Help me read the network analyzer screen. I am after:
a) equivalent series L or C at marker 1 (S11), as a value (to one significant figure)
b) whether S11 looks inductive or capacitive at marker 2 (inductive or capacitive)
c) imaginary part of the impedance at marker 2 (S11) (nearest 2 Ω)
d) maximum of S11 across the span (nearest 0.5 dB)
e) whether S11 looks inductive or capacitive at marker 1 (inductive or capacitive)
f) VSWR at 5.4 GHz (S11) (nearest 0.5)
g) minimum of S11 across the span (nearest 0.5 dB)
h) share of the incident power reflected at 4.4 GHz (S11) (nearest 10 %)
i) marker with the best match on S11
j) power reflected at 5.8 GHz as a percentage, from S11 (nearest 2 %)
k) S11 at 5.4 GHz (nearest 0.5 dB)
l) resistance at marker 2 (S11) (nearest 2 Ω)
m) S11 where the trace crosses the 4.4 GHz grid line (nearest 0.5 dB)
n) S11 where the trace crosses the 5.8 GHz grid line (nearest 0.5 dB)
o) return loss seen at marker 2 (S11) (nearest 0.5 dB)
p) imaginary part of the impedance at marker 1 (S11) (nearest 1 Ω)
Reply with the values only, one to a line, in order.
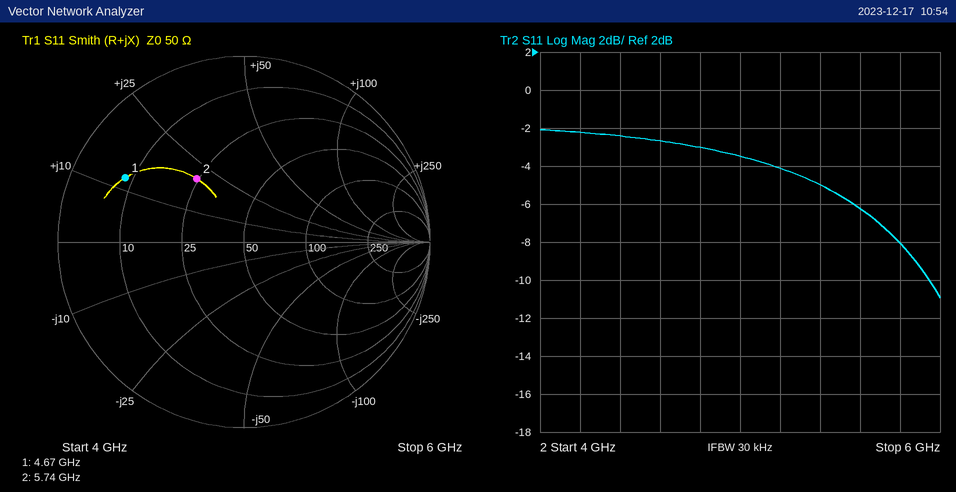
400 pH
inductive
+20 Ω
-2.0 dB
inductive
3.5
-11.0 dB
60 %
marker 2
16 %
-5.0 dB
24 Ω
-2.5 dB
-8.0 dB
7.5 dB
+12 Ω
